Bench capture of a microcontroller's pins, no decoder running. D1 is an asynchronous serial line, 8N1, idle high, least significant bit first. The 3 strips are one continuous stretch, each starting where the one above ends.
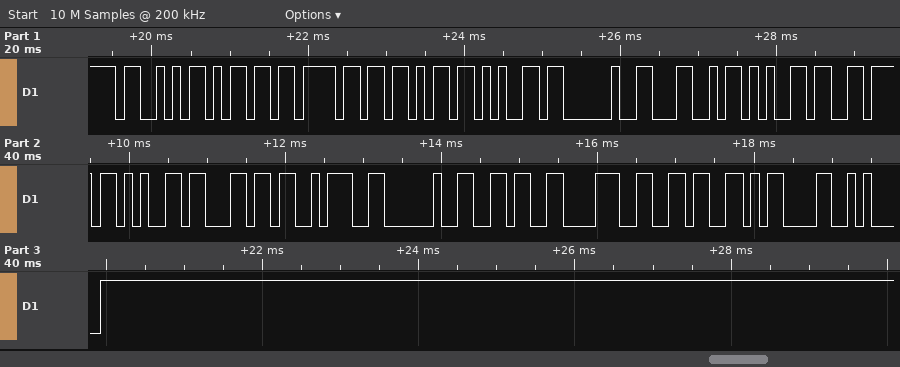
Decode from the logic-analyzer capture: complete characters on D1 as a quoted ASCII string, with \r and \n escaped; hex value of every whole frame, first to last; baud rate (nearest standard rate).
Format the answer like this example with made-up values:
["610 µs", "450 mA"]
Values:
["\"Smoke Level: 686\\r\\n\"", "0x53 0x6D 0x6F 0x6B 0x65 0x20 0x4C 0x65 0x76 0x65 0x6C 0x3A 0x20 0x36 0x38 0x36 0x0D 0x0A", "9600 baud"]
